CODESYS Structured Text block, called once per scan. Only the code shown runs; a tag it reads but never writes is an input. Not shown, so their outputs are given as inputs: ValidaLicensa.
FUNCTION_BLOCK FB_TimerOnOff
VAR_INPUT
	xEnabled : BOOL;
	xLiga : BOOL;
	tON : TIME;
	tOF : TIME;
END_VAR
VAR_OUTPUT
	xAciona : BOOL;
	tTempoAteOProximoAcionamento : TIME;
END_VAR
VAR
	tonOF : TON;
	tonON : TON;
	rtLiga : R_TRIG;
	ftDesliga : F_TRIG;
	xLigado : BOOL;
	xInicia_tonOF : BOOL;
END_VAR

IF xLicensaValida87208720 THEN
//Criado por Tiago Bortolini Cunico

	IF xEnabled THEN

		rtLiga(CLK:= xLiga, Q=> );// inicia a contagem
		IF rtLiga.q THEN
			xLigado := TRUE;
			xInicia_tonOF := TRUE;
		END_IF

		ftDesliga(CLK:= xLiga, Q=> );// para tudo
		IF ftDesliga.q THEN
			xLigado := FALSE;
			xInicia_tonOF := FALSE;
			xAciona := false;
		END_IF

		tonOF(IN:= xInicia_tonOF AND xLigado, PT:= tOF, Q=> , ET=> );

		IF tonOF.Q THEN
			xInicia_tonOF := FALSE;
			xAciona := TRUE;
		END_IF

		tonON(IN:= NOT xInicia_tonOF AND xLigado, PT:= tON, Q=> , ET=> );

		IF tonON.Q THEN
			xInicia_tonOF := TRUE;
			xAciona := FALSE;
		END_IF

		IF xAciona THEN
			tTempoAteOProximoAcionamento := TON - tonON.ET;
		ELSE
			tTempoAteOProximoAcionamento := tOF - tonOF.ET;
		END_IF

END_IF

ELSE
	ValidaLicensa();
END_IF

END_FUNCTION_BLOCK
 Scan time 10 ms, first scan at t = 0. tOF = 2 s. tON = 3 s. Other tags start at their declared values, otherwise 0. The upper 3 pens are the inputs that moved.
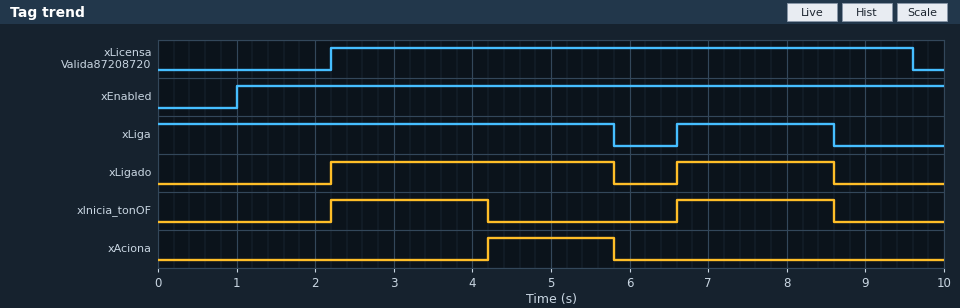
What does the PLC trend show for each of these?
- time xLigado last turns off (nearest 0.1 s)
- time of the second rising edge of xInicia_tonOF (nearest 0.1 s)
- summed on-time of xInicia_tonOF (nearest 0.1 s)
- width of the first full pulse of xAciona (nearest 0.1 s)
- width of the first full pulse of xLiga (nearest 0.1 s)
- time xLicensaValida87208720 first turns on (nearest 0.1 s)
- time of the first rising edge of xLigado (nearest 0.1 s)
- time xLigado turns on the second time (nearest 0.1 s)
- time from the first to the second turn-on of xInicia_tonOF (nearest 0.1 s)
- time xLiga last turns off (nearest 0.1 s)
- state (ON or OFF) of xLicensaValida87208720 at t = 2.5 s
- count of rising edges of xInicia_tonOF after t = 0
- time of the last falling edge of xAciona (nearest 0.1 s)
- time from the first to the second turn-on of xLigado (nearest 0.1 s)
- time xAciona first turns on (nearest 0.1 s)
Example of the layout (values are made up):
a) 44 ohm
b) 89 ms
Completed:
a) 8.6 s
b) 6.6 s
c) 4.0 s
d) 1.6 s
e) 2.0 s
f) 2.2 s
g) 2.2 s
h) 6.6 s
i) 4.4 s
j) 8.6 s
k) ON
l) 2
m) 5.8 s
n) 4.4 s
o) 4.2 s
